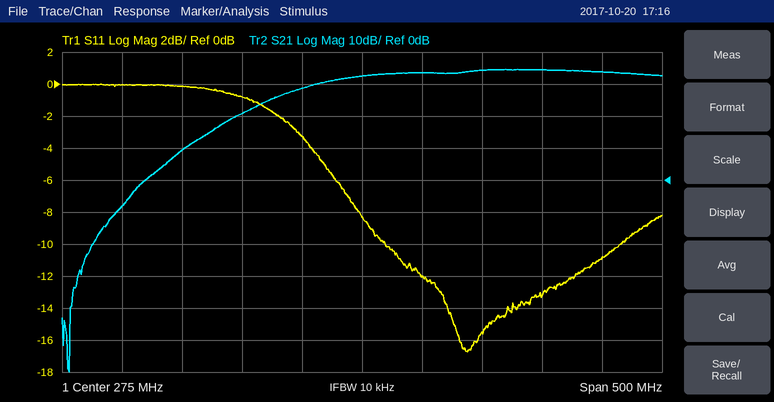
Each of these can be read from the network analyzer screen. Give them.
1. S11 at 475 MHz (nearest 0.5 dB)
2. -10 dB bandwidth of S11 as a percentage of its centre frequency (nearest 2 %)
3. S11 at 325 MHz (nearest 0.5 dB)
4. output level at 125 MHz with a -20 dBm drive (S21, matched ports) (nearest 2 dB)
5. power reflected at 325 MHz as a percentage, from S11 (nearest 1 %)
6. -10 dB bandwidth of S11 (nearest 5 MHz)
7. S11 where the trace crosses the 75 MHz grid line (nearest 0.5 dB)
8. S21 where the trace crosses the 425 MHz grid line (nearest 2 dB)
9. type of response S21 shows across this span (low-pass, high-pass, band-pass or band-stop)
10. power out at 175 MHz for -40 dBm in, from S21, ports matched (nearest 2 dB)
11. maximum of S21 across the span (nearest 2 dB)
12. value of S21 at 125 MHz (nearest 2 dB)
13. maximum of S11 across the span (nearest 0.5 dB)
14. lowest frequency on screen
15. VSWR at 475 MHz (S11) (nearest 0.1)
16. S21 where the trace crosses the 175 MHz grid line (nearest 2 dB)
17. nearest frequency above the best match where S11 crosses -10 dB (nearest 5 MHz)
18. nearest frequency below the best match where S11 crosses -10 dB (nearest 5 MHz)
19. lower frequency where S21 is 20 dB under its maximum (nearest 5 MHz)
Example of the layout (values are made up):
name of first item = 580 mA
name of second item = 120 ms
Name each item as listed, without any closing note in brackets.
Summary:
S11 at 475 MHz = -11.0 dB
-10 dB bandwidth of S11 as a percentage of its centre frequency = 50 %
S11 at 325 MHz = -12.0 dB
output level at 125 MHz with a -20 dBm drive (S21, matched ports) = -10 dBm
power reflected at 325 MHz as a percentage, from S11 = 6 %
-10 dB bandwidth of S11 = 195 MHz
S11 where the trace crosses the 75 MHz grid line = 0.0 dB
S21 where the trace crosses the 425 MHz grid line = 34 dB
type of response S21 shows across this span = high-pass
power out at 175 MHz for -40 dBm in, from S21, ports matched = -20 dBm
maximum of S21 across the span = 34 dB
value of S21 at 125 MHz = 10 dB
maximum of S11 across the span = 0.0 dB
lowest frequency on screen = 25 MHz
VSWR at 475 MHz (S11) = 1.8
S21 where the trace crosses the 175 MHz grid line = 20 dB
nearest frequency above the best match where S11 crosses -10 dB = 490 MHz
nearest frequency below the best match where S11 crosses -10 dB = 295 MHz
lower frequency where S21 is 20 dB under its maximum = 145 MHz
